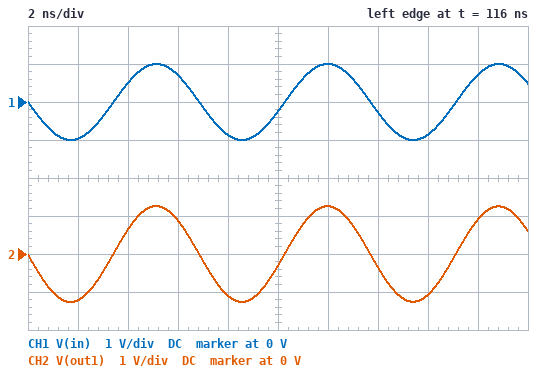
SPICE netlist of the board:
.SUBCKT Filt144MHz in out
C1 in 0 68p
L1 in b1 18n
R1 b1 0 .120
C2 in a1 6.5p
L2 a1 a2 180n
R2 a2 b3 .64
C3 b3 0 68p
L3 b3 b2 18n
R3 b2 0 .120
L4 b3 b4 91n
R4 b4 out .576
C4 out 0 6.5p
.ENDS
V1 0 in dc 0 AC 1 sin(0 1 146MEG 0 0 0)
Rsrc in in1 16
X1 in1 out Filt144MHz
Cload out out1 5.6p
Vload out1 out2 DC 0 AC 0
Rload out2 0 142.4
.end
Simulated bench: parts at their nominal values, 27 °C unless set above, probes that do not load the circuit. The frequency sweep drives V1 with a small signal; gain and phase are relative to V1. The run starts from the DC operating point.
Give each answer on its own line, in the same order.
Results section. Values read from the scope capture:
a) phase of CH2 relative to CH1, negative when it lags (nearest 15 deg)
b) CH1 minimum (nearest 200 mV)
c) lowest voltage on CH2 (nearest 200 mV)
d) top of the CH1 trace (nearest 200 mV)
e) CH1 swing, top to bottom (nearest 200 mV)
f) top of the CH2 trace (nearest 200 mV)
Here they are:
0 deg
-1.0 V
-1.2 V
1.0 V
2.0 V
1.2 V
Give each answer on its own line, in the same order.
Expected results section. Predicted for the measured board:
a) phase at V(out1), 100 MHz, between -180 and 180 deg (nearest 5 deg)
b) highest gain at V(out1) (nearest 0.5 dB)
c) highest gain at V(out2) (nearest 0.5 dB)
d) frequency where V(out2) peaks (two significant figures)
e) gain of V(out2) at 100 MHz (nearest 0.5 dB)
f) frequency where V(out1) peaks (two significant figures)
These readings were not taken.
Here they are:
75 deg
3.0 dB
3.0 dB
150 MHz
-15.5 dB
150 MHz
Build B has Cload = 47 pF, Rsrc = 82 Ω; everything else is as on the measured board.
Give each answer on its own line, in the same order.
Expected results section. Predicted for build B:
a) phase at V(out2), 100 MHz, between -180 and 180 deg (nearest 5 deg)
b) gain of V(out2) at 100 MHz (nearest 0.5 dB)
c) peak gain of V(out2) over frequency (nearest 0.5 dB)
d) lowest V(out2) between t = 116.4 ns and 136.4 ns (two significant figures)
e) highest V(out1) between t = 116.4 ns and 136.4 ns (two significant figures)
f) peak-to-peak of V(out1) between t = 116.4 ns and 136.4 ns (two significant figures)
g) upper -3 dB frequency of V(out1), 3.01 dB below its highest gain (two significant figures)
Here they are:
35 deg
-22.0 dB
-4.0 dB
-630 mV
630 mV
1.3 V
190 MHz
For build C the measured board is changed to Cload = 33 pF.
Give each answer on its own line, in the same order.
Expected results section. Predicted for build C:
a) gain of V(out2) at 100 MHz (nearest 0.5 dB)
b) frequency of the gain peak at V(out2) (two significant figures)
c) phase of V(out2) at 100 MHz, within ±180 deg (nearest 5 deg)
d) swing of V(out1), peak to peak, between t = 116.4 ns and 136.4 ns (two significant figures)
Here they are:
-13.0 dB
170 MHz
0 deg
2.3 V
